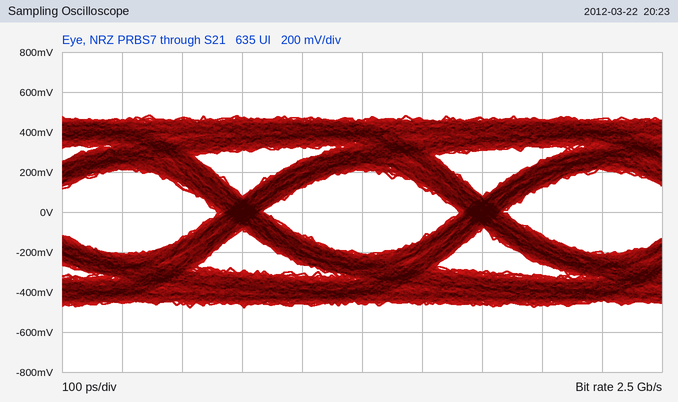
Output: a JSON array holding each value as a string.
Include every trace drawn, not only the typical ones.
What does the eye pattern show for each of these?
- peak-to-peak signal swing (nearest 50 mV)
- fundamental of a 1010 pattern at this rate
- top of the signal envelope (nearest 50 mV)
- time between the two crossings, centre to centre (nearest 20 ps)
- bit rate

["950 mV", "1.25 GHz", "500 mV", "400 ps", "2.5 Gb/s"]
